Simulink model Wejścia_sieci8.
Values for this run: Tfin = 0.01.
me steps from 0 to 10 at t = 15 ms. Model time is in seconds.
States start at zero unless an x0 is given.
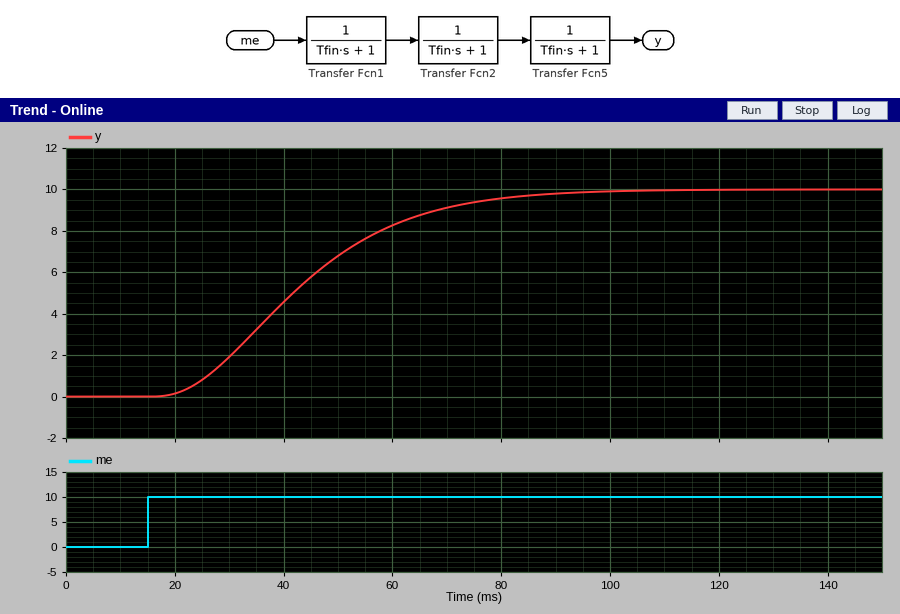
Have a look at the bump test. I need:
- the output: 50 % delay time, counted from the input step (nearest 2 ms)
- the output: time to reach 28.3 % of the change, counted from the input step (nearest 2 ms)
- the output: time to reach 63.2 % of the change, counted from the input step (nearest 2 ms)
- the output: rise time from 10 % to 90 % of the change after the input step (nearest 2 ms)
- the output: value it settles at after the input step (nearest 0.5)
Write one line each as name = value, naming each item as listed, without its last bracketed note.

the output: 50 % delay time, counted from the input step = 26 ms
the output: time to reach 28.3 % of the change, counted from the input step = 18 ms
the output: time to reach 63.2 % of the change, counted from the input step = 32 ms
the output: rise time from 10 % to 90 % of the change after the input step = 42 ms
the output: value it settles at after the input step = 10.0
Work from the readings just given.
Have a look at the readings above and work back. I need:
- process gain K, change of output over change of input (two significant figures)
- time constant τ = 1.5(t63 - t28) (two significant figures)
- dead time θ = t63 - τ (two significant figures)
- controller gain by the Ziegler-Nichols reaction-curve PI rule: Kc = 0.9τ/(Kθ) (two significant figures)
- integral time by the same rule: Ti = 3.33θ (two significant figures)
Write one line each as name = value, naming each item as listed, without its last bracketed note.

process gain K, change of output over change of input = 1.0
time constant τ = 1.5(t63 - t28) = 21 ms
dead time θ = t63 - τ = 11 ms
controller gain by the Ziegler-Nichols reaction-curve PI rule: Kc = 0.9τ/(Kθ) = 1.7
integral time by the same rule: Ti = 3.33θ = 37 ms
